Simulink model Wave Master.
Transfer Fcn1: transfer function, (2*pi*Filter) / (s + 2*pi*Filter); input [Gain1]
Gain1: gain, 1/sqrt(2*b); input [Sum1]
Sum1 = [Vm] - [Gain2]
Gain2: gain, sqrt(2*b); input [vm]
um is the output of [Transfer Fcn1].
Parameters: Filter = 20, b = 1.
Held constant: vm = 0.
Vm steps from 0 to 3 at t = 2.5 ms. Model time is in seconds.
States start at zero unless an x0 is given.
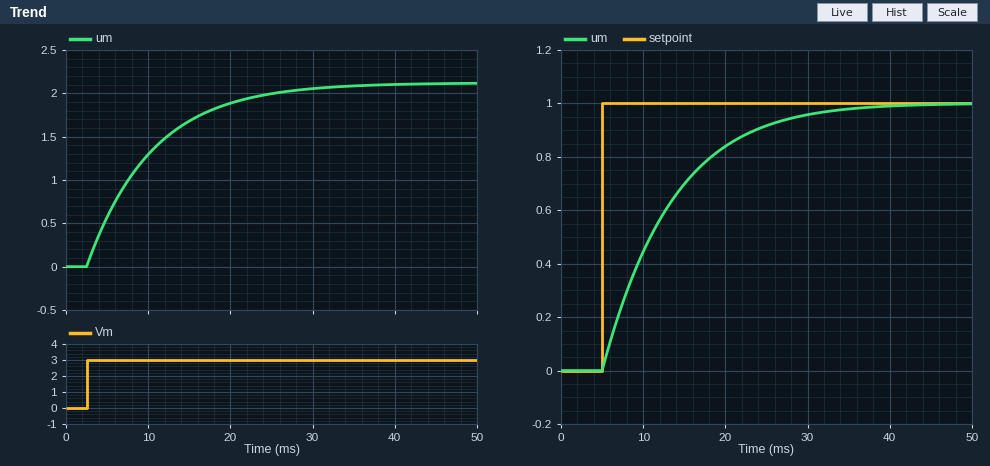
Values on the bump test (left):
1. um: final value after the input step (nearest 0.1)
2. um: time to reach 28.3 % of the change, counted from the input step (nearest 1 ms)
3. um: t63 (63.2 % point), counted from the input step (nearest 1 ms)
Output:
2.1
3 ms
8 ms
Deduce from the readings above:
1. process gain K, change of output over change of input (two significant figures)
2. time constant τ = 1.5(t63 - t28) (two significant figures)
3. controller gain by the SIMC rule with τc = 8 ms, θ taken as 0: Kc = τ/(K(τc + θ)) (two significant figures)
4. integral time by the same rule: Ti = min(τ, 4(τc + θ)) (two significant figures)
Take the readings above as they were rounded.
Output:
0.70
7.5 ms
1.3
7.5 ms
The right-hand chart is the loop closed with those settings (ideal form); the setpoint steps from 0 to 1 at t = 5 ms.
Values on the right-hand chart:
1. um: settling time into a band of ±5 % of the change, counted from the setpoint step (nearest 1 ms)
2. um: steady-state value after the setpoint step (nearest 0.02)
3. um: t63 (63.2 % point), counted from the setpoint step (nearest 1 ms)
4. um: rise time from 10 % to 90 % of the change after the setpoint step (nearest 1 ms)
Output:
24 ms
1.00
8 ms
18 ms
